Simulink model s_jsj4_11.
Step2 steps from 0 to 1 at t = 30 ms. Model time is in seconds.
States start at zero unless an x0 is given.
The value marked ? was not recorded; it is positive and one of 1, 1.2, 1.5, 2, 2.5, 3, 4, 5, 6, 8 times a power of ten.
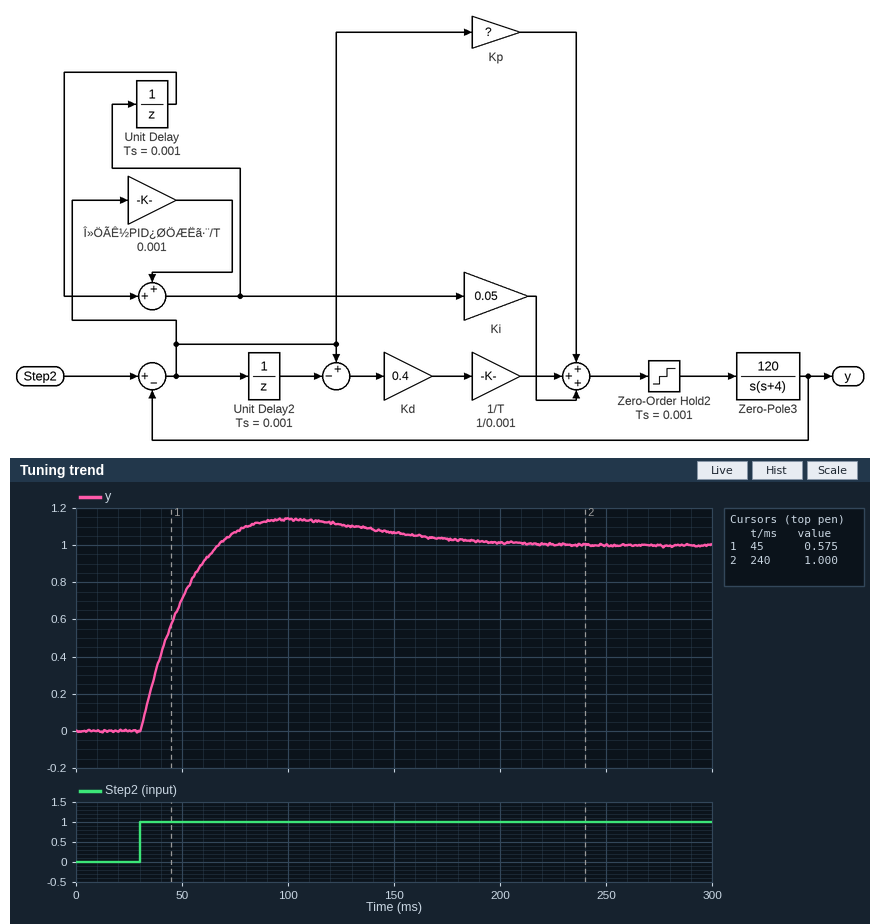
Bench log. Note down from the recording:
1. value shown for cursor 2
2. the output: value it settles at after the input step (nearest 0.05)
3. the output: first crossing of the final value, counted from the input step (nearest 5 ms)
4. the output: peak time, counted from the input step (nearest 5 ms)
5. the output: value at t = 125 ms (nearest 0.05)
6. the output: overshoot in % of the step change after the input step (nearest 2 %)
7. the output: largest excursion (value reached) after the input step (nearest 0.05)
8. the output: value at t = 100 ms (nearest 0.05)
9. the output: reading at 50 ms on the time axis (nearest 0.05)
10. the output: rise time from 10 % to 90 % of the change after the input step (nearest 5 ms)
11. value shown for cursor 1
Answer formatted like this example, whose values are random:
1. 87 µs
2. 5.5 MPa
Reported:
1. 1.000
2. 1.00
3. 35 ms
4. 70 ms
5. 1.10
6. 14 %
7. 1.15
8. 1.15
9. 0.70
10. 25 ms
11. 0.575
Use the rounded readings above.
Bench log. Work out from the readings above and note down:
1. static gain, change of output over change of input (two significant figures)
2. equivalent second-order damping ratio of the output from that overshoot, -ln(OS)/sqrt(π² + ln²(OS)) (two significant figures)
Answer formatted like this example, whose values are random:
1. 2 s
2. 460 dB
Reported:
1. 1.0
2. 0.53
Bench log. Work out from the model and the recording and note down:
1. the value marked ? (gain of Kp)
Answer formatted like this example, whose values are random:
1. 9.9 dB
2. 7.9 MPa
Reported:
1. 8
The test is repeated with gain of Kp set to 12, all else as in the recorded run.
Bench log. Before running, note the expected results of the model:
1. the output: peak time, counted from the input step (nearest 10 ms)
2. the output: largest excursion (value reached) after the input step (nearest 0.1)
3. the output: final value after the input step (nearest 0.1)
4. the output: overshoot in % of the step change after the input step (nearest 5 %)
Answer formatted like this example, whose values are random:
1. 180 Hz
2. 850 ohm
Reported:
1. 60 ms
2. 1.2
3. 1.0
4. 20 %
